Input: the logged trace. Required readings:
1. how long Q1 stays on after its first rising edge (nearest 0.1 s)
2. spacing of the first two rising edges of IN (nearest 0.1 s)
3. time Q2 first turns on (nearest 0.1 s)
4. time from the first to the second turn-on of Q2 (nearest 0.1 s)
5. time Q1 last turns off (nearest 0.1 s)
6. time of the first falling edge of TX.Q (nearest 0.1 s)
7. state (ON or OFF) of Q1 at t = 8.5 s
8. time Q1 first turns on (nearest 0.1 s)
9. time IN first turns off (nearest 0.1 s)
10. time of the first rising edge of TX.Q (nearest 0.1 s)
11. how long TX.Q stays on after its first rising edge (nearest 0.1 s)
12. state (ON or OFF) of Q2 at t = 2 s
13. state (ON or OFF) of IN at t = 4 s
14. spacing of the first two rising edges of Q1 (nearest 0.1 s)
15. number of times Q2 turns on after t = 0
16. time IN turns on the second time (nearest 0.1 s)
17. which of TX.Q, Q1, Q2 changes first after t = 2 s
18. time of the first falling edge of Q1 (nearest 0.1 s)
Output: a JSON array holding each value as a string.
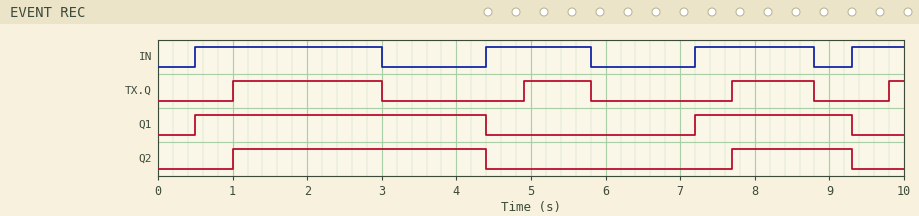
["3.9 s", "3.9 s", "1.0 s", "6.7 s", "9.3 s", "3.0 s", "ON", "0.5 s", "3.0 s", "1.0 s", "2.0 s", "ON", "OFF", "6.7 s", "2", "4.4 s", "TX.Q", "4.4 s"]
